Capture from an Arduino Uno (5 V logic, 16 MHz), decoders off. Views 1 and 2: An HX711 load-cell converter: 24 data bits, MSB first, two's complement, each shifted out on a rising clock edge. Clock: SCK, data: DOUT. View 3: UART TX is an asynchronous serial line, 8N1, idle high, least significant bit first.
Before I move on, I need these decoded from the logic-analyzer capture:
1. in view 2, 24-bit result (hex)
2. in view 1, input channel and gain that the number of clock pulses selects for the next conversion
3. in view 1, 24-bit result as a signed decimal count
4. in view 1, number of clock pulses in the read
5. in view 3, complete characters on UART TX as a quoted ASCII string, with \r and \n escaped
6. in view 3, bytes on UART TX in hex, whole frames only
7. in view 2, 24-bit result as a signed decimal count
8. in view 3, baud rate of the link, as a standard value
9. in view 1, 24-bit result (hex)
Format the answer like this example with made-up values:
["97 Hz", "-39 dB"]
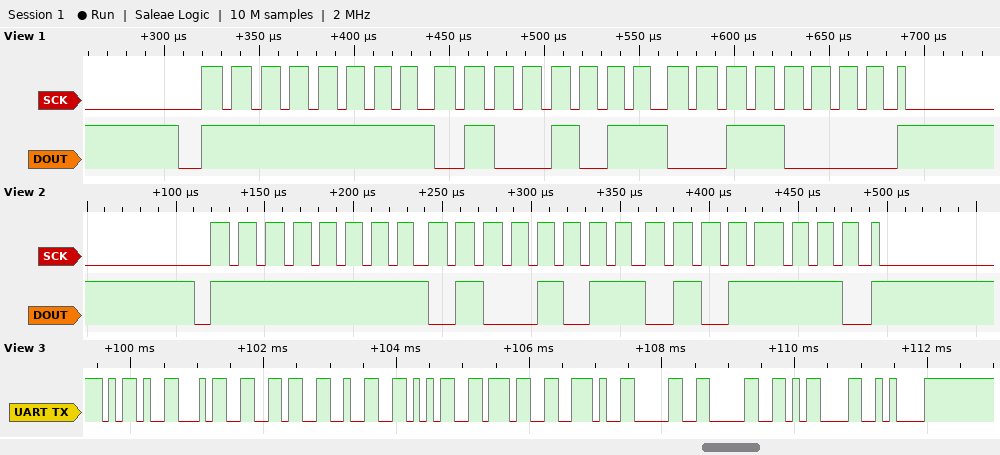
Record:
["0xFF4B5E", "channel A, gain 128", "-46288", "25", "\"-46257.00\\r\\n\"", "2D 34 36 32 35 37 2E 30 30 0D 0A", "-46242", "9600 baud", "0xFF4B30"]
